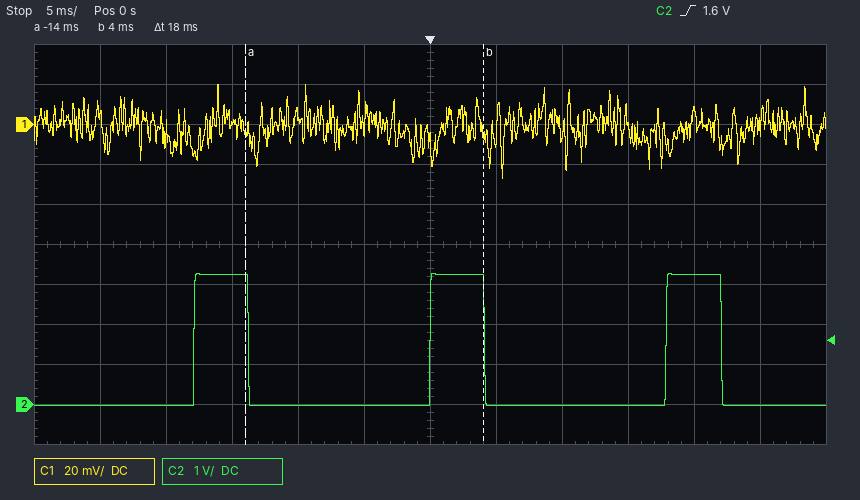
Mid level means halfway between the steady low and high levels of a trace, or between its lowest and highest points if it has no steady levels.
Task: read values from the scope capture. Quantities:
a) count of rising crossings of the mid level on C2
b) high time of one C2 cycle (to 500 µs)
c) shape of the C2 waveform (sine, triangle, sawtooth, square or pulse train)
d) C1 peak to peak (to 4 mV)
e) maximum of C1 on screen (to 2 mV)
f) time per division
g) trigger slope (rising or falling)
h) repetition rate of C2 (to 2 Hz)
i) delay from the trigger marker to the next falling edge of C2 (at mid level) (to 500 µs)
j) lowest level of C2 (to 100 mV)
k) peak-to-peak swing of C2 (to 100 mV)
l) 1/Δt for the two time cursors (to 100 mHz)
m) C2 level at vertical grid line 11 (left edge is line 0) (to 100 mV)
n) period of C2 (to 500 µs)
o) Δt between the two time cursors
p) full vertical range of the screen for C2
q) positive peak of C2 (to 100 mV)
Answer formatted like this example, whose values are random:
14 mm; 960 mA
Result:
3; 4.0 ms; pulse train; 48 mV; 20 mV; 5 ms; rising; 56 Hz; 4.0 ms; 0.0 V; 3.3 V; 55.6 Hz; 0.0 V; 18.0 ms; 18 ms; 10 V; 3.3 V
